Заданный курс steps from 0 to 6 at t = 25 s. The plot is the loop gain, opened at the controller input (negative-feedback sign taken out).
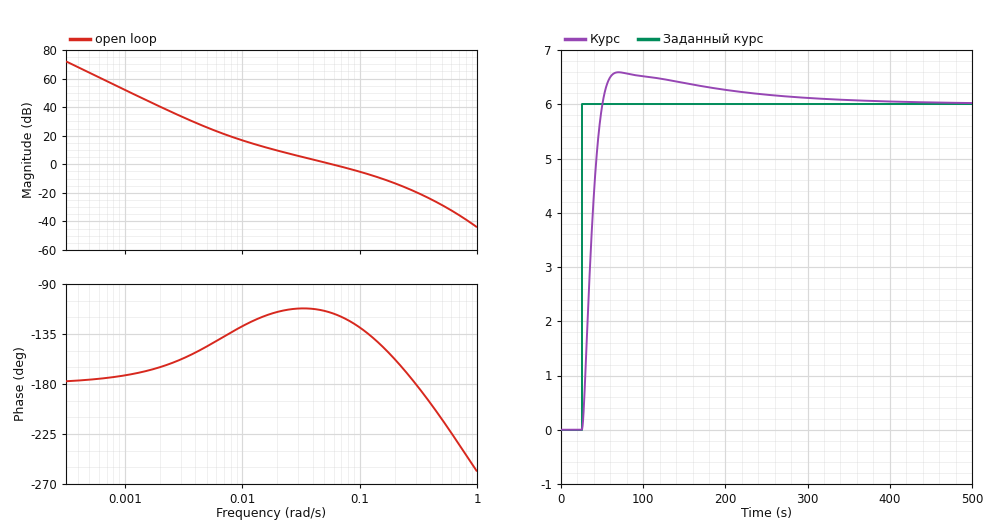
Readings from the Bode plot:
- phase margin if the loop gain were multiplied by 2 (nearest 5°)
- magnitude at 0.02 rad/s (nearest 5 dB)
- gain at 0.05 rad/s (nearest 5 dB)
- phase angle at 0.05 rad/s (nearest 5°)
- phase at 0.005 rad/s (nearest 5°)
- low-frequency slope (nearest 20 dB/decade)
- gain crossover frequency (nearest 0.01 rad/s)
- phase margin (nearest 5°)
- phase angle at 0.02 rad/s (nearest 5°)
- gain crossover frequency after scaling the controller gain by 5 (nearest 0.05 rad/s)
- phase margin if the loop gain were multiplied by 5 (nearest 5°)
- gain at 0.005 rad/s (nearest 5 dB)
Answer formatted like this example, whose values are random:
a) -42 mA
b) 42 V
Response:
a) 50°
b) 10 dB
c) 0 dB
d) -115°
e) -145°
f) -40 dB/decade
g) 0.06 rad/s
h) 65°
i) -115°
j) 0.20 rad/s
k) 20°
l) 25 dB
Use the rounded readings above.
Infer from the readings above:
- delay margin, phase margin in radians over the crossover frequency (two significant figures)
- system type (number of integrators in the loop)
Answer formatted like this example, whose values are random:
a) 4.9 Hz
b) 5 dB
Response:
a) 19 s
b) 2
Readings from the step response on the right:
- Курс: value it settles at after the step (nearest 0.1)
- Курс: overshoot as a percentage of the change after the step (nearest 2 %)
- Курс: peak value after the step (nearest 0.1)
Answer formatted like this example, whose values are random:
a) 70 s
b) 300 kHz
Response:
a) 6.0
b) 10 %
c) 6.6
